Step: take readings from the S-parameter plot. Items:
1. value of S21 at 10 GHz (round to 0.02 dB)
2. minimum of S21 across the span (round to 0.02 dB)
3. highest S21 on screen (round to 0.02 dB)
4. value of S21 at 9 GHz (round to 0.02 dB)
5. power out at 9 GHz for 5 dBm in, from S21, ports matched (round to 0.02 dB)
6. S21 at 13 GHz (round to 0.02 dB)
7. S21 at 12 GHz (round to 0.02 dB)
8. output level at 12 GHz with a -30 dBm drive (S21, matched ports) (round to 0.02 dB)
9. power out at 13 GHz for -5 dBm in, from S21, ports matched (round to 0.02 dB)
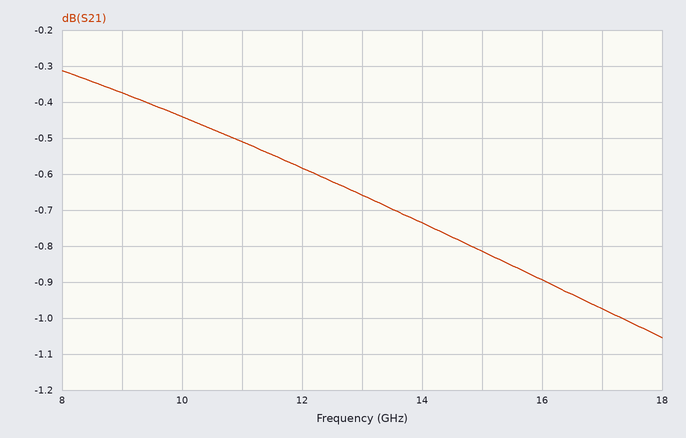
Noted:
-0.44 dB
-1.06 dB
-0.32 dB
-0.38 dB
4.62 dBm
-0.66 dB
-0.58 dB
-30.58 dBm
-5.66 dBm
